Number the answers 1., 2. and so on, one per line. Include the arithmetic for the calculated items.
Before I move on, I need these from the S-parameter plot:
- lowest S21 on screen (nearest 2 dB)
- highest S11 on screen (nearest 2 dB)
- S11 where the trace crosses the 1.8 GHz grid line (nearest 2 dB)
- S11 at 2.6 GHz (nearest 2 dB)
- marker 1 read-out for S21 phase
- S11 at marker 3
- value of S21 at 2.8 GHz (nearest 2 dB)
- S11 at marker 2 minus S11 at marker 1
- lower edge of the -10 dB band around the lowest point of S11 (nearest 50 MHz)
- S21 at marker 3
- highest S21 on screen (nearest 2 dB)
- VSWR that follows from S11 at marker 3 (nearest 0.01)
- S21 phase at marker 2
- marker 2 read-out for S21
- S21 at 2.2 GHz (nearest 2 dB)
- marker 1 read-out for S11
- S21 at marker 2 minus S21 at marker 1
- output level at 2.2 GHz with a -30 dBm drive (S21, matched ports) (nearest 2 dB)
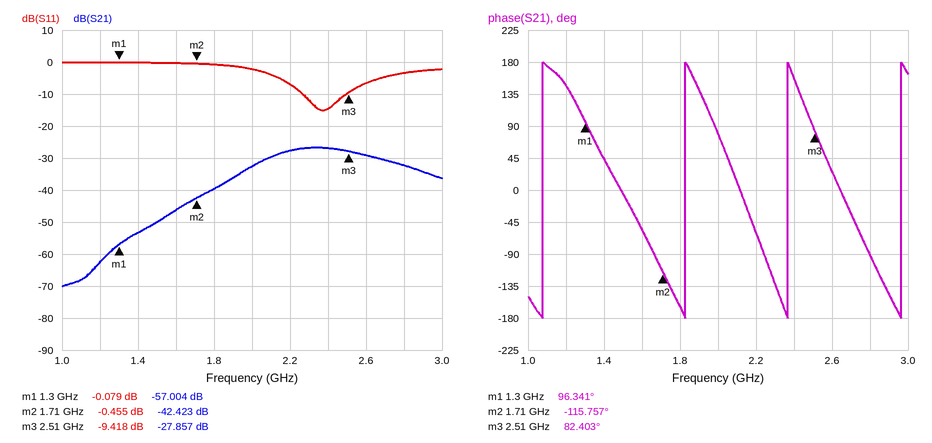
1. -70 dB
2. 0 dB
3. 0 dB
4. -6 dB
5. 96.341°
6. -9.418 dB
7. -32 dB
8. -0.455 − (-0.079) = -0.376 dB
9. 2.25 GHz
10. -27.857 dB
11. -26 dB
12. (1 + 0.3381)/(1 − 0.3381) ≈ 2.02
13. -115.757°
14. -42.423 dB
15. -28 dB
16. -0.079 dB
17. -42.423 − (-57.004) = 14.581 dB
18. -30 dBm + (-28 dB) = -58 dBm
